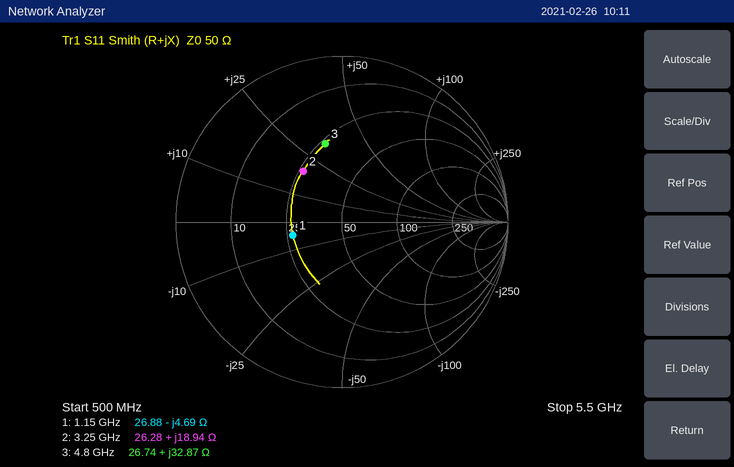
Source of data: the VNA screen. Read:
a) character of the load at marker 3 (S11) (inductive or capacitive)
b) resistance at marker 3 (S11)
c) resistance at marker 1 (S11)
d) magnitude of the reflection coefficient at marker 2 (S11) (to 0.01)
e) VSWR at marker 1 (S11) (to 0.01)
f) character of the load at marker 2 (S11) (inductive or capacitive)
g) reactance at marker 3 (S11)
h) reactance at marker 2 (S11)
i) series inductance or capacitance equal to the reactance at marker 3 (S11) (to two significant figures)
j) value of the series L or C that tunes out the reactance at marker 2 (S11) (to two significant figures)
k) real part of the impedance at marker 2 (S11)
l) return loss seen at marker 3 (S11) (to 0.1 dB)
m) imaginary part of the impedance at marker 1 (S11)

inductive
26.74 Ω
26.88 Ω
0.39
1.88
inductive
+32.87 Ω
+18.94 Ω
1.1 nH
2.6 pF
26.28 Ω
6.3 dB
-4.69 Ω
